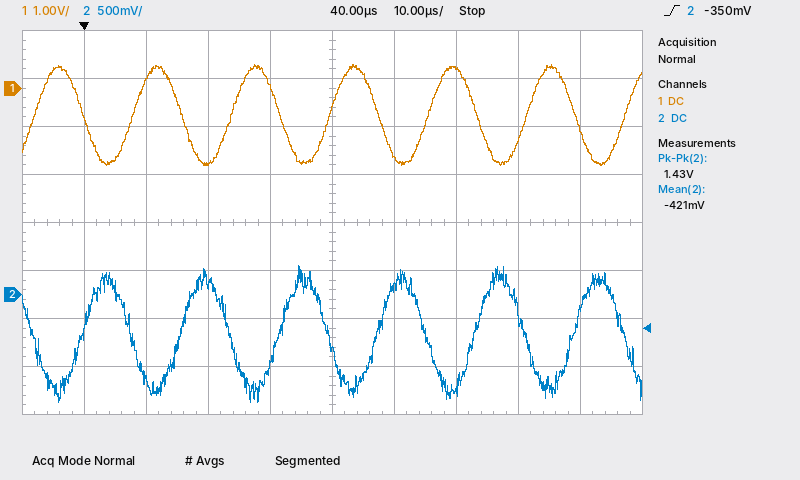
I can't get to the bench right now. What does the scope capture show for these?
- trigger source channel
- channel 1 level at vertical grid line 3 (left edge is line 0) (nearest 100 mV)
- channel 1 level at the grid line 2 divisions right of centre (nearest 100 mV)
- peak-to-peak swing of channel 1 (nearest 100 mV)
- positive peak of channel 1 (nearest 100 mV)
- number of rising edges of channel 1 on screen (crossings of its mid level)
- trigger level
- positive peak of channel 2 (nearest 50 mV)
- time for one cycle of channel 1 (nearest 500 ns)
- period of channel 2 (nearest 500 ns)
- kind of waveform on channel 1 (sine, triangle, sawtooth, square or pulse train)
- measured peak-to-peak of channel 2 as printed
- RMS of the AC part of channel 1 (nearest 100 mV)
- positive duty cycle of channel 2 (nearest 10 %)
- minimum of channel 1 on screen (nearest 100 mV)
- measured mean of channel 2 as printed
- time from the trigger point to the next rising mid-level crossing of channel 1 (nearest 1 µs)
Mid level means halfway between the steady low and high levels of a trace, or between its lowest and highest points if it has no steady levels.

channel 2
-1.6 V
400 mV
2.1 V
500 mV
7
-350 mV
300 mV
16.0 µs
16.0 µs
sine
1.43 V
700 mV
50 %
-1.6 V
-421 mV
8 µs
